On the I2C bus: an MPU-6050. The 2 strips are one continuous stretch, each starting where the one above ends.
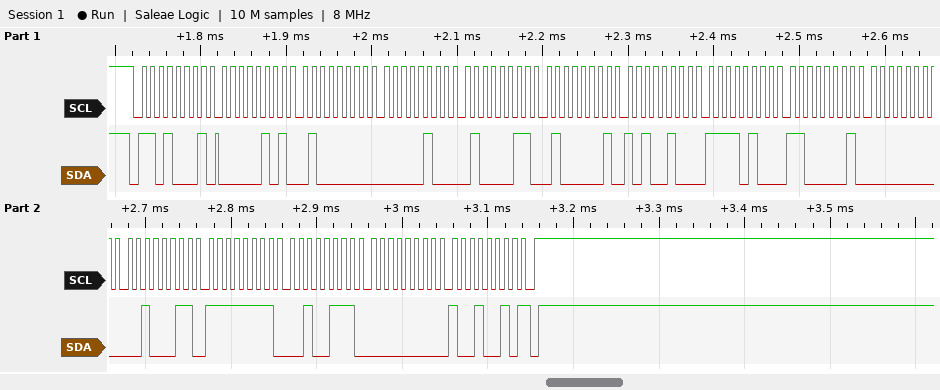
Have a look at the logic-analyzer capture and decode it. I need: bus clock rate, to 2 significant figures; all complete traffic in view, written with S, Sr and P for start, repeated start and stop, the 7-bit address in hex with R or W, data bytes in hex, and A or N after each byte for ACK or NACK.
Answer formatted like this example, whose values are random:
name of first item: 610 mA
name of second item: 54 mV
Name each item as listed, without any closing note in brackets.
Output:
bus clock rate, to 2 significant figures: 100 kHz
all complete traffic in view, written with S, Sr and P for start, repeated start and stop, the 7-bit address in hex with R or W, data bytes in hex, and A or N after each byte for ACK or NACK: S 68R A 05 A 40 A 04 A 43 A 41 A A4 A F4 A C1 A 00 A 23 A FF A 27 A 00 A 92 N P
